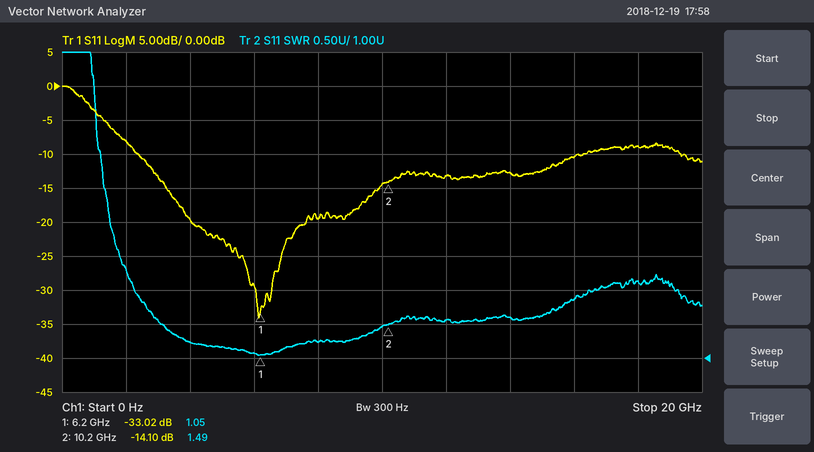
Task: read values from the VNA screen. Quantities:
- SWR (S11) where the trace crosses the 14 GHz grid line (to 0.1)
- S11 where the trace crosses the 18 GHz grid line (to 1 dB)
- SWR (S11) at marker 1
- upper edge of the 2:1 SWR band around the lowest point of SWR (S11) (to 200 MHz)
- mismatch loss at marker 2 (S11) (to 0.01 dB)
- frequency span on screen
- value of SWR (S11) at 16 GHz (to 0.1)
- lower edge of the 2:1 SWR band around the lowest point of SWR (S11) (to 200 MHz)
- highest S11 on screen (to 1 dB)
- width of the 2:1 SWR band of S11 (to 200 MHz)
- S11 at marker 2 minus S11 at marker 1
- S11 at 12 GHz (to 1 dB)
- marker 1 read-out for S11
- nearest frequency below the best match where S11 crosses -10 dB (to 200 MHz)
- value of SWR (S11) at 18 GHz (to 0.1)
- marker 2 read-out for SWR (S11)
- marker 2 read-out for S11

1.6
-9 dB
1.05
16.6 GHz
0.17 dB
20 GHz
1.9
2.2 GHz
0 dB
14.4 GHz
18.92 dB
-13 dB
-33.02 dB
2.4 GHz
2.1
1.49
-14.10 dB
